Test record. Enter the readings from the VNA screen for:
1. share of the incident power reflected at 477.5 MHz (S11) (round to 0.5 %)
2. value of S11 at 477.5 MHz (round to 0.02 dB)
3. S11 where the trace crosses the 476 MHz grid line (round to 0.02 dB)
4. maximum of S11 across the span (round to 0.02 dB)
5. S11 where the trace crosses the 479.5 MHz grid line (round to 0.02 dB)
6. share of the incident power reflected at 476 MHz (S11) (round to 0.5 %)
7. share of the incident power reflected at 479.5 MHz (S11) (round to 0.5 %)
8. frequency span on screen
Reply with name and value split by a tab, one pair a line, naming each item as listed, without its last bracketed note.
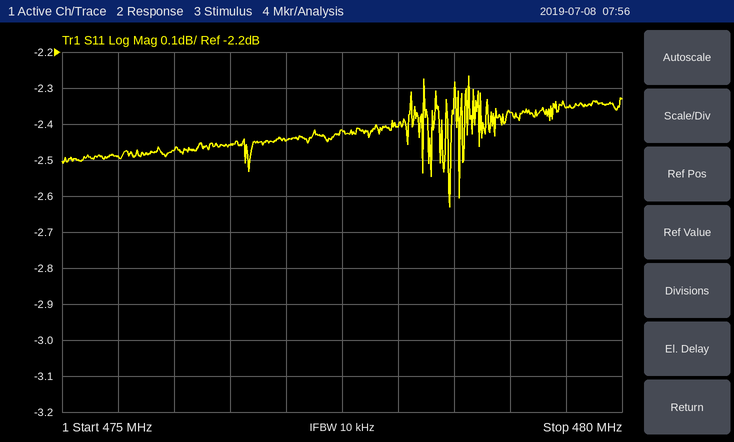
share of the incident power reflected at 477.5 MHz (S11)	57.5 %
value of S11 at 477.5 MHz	-2.42 dB
S11 where the trace crosses the 476 MHz grid line	-2.48 dB
maximum of S11 across the span	-2.26 dB
S11 where the trace crosses the 479.5 MHz grid line	-2.36 dB
share of the incident power reflected at 476 MHz (S11)	56.5 %
share of the incident power reflected at 479.5 MHz (S11)	58.0 %
frequency span on screen	5 MHz
